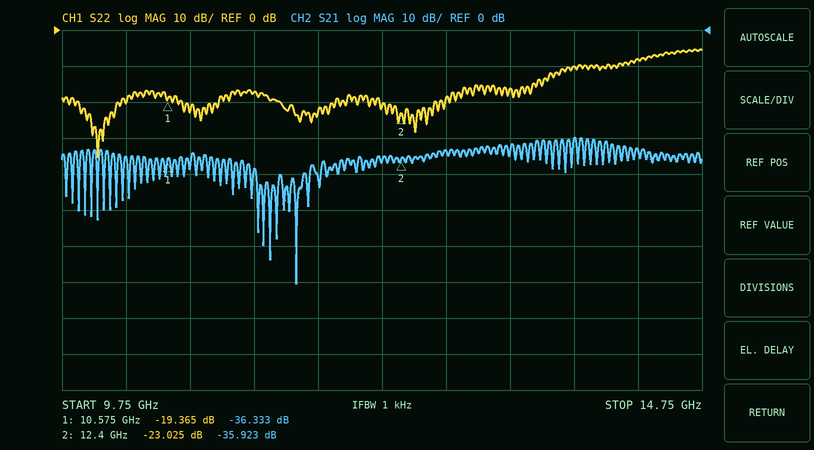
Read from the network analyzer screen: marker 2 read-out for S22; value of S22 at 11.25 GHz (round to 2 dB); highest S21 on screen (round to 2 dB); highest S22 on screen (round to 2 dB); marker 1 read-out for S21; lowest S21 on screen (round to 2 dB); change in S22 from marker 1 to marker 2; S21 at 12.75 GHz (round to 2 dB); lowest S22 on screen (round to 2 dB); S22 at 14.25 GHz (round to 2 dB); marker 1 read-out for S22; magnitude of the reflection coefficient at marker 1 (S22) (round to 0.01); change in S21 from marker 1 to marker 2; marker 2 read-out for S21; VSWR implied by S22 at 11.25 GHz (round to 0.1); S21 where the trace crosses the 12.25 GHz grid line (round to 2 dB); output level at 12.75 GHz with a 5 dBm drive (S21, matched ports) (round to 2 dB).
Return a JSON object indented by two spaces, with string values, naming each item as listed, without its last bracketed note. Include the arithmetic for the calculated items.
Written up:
{
  "marker 2 read-out for S22": "-23.025 dB",
  "value of S22 at 11.25 GHz": "-18 dB",
  "highest S21 on screen": "-30 dB",
  "highest S22 on screen": "-6 dB",
  "marker 1 read-out for S21": "-36.333 dB",
  "lowest S21 on screen": "-70 dB",
  "change in S22 from marker 1 to marker 2": "-23.025 − (-19.365) = -3.660 dB",
  "S21 at 12.75 GHz": "-34 dB",
  "lowest S22 on screen": "-36 dB",
  "S22 at 14.25 GHz": "-8 dB",
  "marker 1 read-out for S22": "-19.365 dB",
  "magnitude of the reflection coefficient at marker 1 (S22)": "10^(-19.365/20) ≈ 0.11",
  "change in S21 from marker 1 to marker 2": "-35.923 − (-36.333) = 0.410 dB",
  "marker 2 read-out for S21": "-35.923 dB",
  "VSWR implied by S22 at 11.25 GHz": "|Γ| = 10^(-18/20) = 0.1259; VSWR = (1 + 0.1259)/(1 − 0.1259) ≈ 1.3",
  "S21 where the trace crosses the 12.25 GHz grid line": "-36 dB",
  "output level at 12.75 GHz with a 5 dBm drive (S21, matched ports)": "5 dBm + (-34 dB) = -28 dBm"
}
